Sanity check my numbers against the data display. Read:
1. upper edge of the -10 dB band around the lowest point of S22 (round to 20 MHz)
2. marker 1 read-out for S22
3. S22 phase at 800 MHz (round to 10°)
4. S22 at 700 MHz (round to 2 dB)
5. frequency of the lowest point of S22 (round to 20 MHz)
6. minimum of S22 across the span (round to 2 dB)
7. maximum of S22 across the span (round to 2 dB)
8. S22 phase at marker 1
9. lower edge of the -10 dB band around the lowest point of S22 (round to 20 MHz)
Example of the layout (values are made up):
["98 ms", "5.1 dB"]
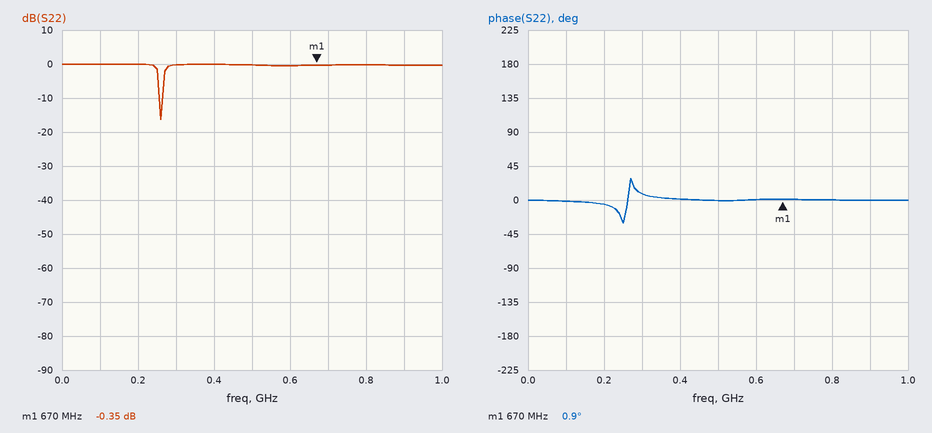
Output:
["260 MHz", "-0.35 dB", "0°", "0 dB", "260 MHz", "-16 dB", "0 dB", "0.9°", "260 MHz"]
